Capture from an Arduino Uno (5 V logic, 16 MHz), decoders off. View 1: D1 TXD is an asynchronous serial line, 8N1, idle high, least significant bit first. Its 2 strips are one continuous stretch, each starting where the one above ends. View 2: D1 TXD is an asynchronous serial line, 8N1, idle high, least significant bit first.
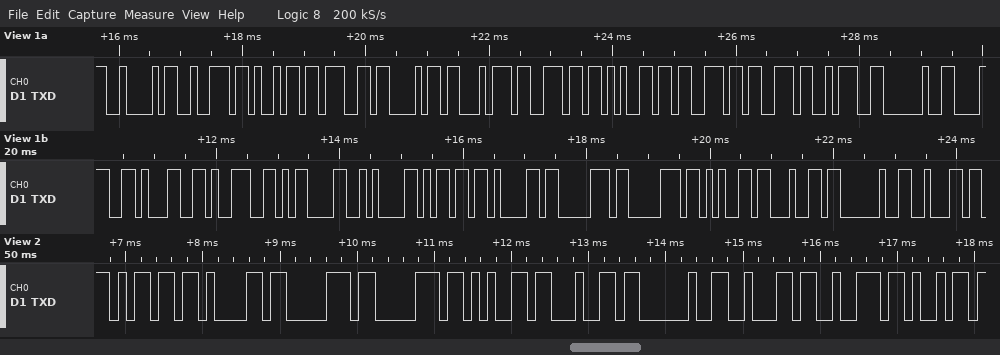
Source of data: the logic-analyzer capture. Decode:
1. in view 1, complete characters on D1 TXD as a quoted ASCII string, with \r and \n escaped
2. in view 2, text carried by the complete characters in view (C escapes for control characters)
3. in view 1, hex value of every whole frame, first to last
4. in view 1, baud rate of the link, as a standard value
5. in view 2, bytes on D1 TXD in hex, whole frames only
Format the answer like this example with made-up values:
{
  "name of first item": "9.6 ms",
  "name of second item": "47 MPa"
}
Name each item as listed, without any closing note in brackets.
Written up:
{
  "in view 1, complete characters on D1 TXD as a quoted ASCII string, with \\r and \\n escaped": "\"Brightness: 819\\r\\nmapped b\"",
  "in view 2, text carried by the complete characters in view": "\"mapped bri\"",
  "in view 1, hex value of every whole frame, first to last": "42 72 69 67 68 74 6E 65 73 73 3A 20 38 31 39 0D 0A 6D 61 70 70 65 64 20 62",
  "in view 1, baud rate of the link, as a standard value": "9600 baud",
  "in view 2, bytes on D1 TXD in hex, whole frames only": "6D 61 70 70 65 64 20 62 72 69"
}
